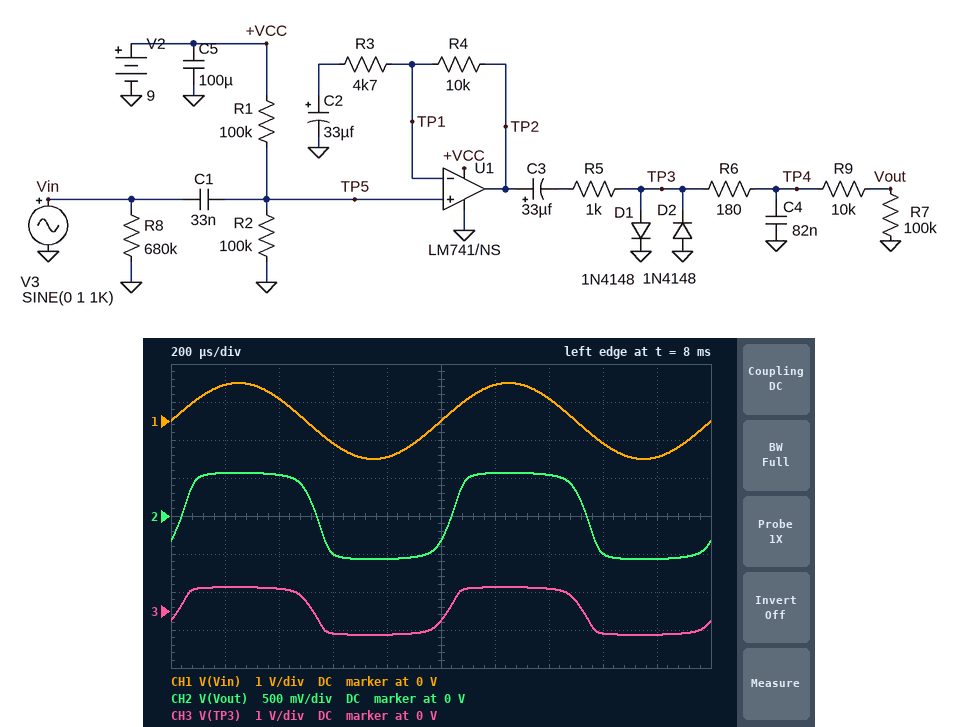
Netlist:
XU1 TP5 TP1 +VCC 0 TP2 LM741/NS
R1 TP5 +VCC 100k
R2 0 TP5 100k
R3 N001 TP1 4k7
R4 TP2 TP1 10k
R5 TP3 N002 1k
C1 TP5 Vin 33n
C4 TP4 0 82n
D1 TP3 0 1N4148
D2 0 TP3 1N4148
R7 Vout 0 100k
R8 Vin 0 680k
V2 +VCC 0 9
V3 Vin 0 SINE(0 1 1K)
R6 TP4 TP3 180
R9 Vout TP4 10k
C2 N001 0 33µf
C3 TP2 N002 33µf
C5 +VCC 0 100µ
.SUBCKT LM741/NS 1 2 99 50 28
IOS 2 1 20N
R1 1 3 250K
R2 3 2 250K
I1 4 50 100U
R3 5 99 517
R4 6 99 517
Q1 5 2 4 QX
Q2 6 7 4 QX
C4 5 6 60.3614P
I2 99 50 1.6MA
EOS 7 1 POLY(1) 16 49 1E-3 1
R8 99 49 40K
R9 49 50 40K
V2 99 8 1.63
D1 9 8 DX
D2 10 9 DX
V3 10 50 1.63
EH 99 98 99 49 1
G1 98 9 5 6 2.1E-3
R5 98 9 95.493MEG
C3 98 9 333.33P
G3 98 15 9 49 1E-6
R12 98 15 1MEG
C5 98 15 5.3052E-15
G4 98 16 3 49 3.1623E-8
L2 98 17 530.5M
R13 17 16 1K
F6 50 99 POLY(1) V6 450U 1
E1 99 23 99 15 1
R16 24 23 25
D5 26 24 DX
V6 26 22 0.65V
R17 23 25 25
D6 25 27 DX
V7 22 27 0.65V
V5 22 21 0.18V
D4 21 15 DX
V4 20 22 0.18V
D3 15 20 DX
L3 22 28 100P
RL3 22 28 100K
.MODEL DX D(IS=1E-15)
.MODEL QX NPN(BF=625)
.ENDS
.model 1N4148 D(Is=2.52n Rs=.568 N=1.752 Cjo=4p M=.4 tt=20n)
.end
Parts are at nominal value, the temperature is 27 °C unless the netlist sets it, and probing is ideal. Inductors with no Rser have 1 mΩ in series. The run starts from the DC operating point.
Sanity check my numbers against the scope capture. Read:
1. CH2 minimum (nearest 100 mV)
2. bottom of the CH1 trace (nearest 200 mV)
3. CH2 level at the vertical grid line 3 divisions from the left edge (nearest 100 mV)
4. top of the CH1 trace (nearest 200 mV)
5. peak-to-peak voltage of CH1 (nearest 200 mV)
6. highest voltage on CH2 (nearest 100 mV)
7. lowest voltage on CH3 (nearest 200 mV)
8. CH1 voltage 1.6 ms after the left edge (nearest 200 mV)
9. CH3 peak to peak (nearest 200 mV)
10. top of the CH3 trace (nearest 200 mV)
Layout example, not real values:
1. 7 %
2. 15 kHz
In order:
1. -600 mV
2. -1.0 V
3. -500 mV
4. 1.0 V
5. 2.0 V
6. 600 mV
7. -600 mV
8. -600 mV
9. 1.2 V
10. 600 mV
